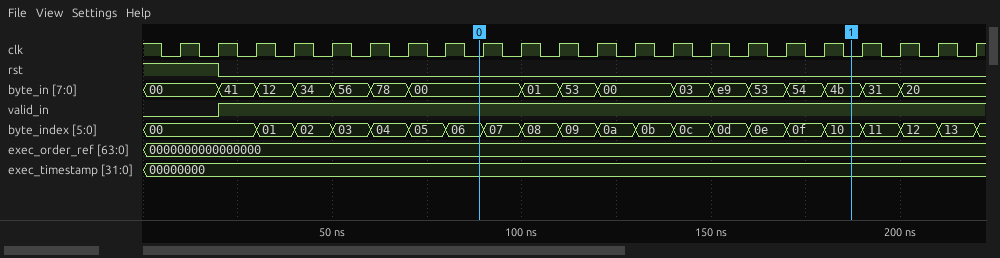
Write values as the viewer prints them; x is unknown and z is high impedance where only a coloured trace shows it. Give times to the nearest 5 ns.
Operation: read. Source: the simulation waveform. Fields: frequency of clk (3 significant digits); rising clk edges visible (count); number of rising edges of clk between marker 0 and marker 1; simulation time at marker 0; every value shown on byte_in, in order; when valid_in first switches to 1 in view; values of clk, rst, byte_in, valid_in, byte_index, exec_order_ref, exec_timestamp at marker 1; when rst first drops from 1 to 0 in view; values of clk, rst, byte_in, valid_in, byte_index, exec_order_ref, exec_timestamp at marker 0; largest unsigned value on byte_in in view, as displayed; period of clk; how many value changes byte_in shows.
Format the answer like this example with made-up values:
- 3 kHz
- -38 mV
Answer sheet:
- 100 MHz
- 22
- 10
- 90 ns
- 00, 41, 12, 34, 56, 78, 00, 01, 53, 00, 03, e9, 53, 54, 4b, 31, 20
- 20 ns
- clk=0, rst=0, byte_in=4b, valid_in=1, byte_index=10, exec_order_ref=0000000000000000, exec_timestamp=00000000
- 20 ns
- clk=0, rst=0, byte_in=00, valid_in=1, byte_index=06, exec_order_ref=0000000000000000, exec_timestamp=00000000
- e9
- 10 ns
- 16
